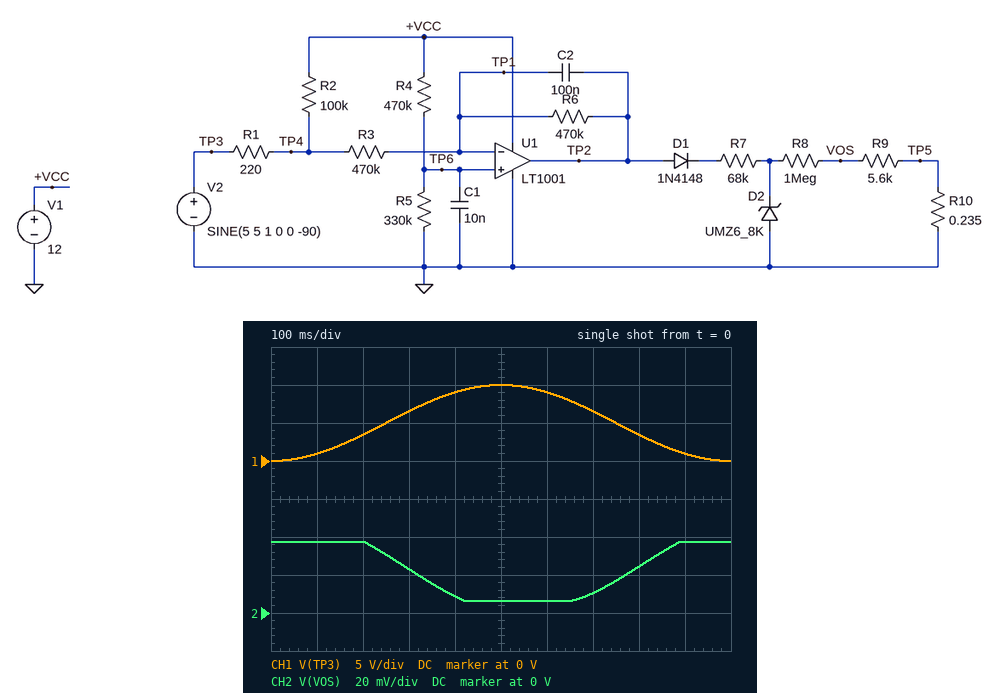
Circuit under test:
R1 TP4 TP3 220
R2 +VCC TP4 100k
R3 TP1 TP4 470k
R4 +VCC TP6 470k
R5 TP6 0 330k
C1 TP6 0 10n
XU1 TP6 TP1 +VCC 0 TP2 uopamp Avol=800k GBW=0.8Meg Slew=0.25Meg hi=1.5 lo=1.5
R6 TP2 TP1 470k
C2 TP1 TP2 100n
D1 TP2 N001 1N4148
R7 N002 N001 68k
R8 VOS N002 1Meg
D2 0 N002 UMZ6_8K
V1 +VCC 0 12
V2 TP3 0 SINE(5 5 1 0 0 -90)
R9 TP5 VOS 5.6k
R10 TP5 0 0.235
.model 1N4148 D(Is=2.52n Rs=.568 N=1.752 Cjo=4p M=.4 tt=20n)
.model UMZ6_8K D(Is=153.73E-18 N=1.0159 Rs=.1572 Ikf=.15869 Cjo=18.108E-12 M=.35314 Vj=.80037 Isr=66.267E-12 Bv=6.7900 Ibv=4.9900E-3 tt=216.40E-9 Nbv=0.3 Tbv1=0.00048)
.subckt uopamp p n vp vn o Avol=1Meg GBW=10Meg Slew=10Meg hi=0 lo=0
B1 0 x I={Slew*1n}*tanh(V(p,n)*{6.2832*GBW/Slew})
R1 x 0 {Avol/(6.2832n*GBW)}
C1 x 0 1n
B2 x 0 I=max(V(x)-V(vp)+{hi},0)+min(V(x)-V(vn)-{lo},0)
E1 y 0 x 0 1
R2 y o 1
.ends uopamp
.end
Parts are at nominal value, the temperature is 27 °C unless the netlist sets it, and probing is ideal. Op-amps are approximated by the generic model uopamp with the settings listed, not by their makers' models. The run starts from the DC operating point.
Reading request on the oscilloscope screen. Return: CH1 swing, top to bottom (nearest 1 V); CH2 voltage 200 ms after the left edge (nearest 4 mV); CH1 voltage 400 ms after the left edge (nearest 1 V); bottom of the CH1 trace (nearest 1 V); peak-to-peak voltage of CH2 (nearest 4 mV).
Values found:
10 V
36 mV
9 V
0 V
32 mV
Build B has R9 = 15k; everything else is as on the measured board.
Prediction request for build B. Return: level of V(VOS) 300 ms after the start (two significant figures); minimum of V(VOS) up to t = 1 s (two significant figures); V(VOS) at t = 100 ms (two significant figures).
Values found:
61 mV
17 mV
100 mV
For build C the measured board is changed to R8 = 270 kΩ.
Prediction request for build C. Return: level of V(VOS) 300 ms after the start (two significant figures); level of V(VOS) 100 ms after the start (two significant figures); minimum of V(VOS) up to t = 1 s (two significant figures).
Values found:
71 mV
140 mV
19 mV
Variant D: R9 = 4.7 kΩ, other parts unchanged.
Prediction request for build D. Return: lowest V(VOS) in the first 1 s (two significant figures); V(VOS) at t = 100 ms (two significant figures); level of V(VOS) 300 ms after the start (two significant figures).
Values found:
5.4 mV
32 mV
19 mV
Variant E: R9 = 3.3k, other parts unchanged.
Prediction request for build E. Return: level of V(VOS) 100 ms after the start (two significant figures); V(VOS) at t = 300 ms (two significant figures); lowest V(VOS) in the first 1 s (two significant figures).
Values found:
22 mV
14 mV
3.8 mV
